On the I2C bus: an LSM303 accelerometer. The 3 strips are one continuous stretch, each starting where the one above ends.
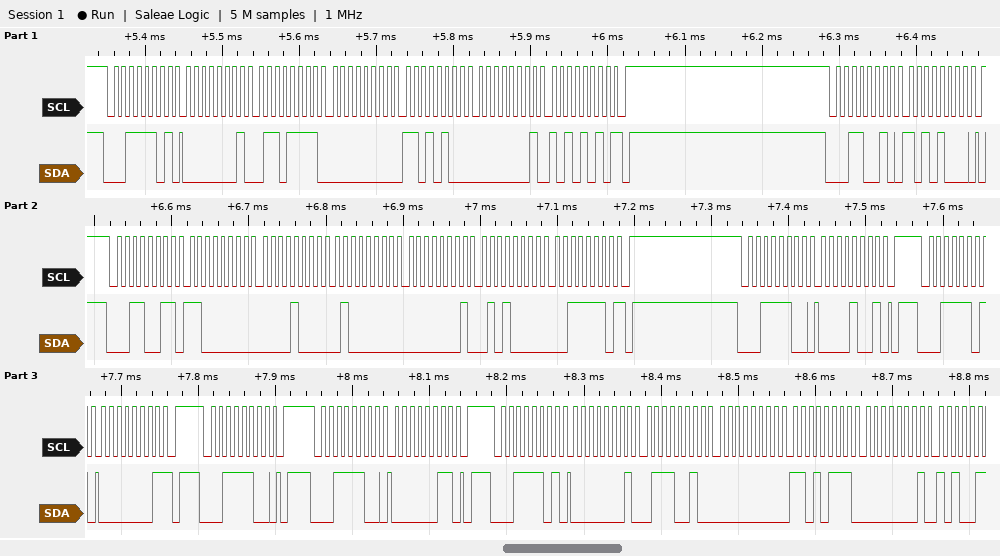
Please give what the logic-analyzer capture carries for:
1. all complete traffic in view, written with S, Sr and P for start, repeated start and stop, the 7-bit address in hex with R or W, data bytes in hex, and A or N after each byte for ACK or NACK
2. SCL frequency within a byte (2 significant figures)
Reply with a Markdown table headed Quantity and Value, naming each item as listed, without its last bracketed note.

| Quantity | Value |
|---|---|
| all complete traffic in view, written with S, Sr and P for start, repeated start and stop, the 7-bit address in hex with R or W, data bytes in hex, and A or N after each byte for ACK or NACK | S 1ER A 01 A 6F A 00 A D4 A 01 A AA N P S 19W A A8 A P S 19R A C0 A 08 A 40 A 01 A 50 A 3E N P S 1EW A 09 A P S 1ER A 01 N P S 1EW A P S 1EW A 03 A P S 1ER A 01 A 72 A 00 A D7 A 01 A |
| SCL frequency within a byte | 100 kHz |
